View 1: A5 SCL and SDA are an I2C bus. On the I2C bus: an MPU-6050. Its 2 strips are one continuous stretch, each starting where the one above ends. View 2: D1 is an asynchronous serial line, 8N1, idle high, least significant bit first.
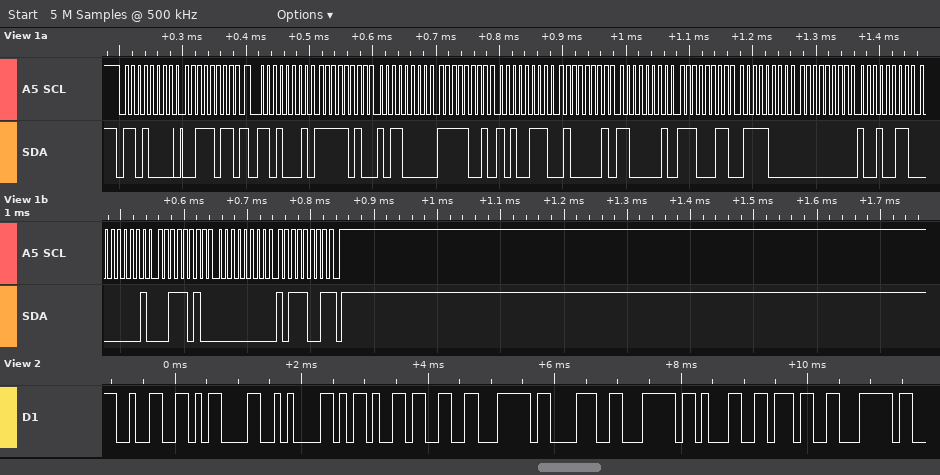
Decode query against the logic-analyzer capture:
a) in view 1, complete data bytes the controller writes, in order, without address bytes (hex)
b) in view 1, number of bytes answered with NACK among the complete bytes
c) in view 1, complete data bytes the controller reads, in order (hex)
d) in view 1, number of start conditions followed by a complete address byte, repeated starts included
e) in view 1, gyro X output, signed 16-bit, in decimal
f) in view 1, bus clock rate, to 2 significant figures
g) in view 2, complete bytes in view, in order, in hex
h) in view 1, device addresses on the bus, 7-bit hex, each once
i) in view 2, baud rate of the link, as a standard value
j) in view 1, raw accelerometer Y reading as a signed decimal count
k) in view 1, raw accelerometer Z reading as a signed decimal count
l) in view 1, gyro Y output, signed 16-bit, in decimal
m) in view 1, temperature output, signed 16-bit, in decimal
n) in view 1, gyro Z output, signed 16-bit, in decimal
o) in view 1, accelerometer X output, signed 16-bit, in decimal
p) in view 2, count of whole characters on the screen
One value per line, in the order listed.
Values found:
3B
1
FA B0 F9 A7 41 C1 E3 78 00 93 01 3A 00 B9
2
147
100 kHz
32 0D 0A 2D 33 7C 38 7C 31 37 7C
0x68
9600 baud
-1625
16833
314
-7304
185
-1360
11
